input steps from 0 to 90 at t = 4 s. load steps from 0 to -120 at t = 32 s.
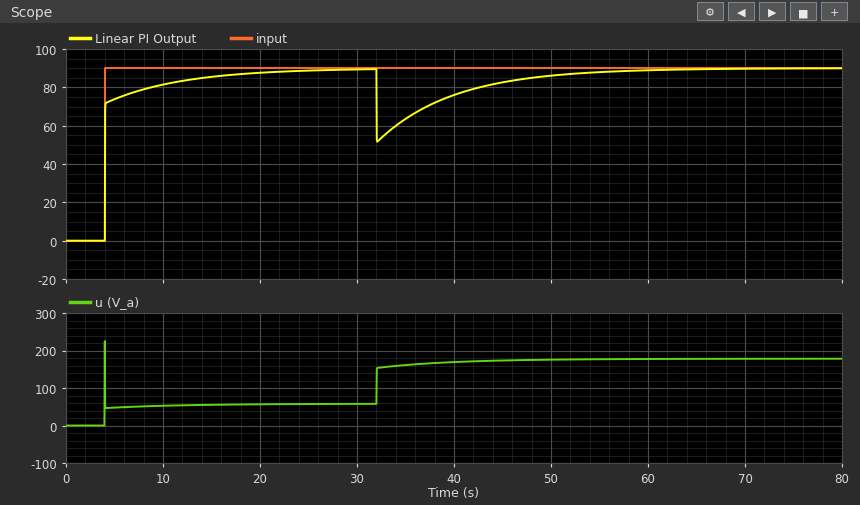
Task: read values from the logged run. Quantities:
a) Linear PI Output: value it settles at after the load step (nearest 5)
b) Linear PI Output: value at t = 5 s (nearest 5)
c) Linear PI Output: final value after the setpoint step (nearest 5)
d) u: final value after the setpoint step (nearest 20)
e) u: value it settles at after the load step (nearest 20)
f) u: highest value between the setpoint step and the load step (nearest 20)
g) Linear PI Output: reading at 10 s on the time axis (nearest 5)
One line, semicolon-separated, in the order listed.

90; 75; 90; 60; 180; 220; 80
